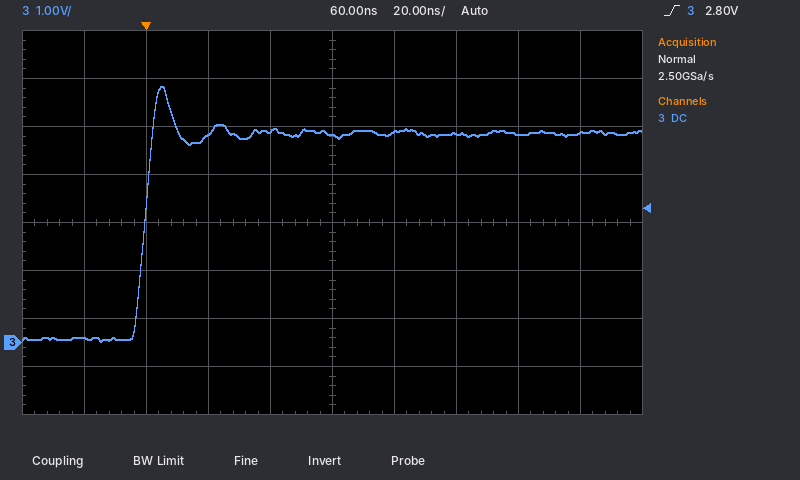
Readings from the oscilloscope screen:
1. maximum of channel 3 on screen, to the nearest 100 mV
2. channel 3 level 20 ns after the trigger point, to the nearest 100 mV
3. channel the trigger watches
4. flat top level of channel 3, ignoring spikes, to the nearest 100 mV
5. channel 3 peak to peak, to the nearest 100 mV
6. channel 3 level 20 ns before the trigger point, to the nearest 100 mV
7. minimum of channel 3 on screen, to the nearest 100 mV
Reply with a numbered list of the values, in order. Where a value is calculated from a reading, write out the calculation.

1. 5.3 V
2. 4.3 V
3. channel 3
4. 4.4 V
5. 5.3 V − (0.0 V) = 5.3 V
6. 100 mV
7. 0.0 V
